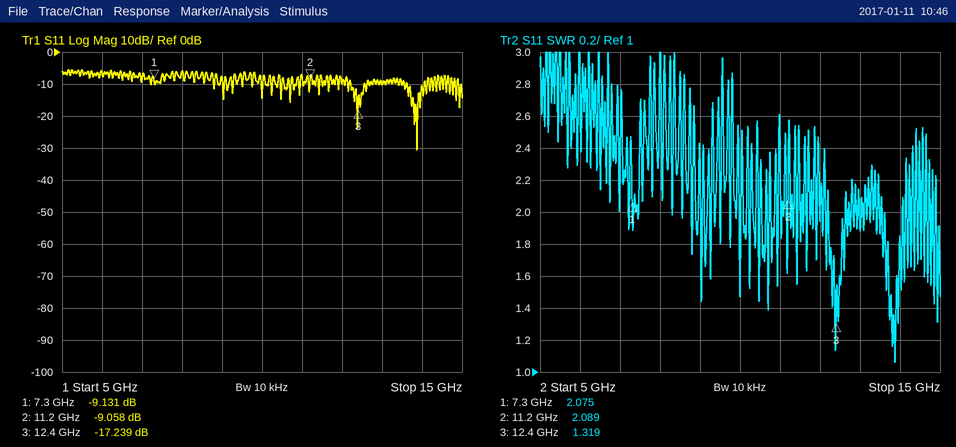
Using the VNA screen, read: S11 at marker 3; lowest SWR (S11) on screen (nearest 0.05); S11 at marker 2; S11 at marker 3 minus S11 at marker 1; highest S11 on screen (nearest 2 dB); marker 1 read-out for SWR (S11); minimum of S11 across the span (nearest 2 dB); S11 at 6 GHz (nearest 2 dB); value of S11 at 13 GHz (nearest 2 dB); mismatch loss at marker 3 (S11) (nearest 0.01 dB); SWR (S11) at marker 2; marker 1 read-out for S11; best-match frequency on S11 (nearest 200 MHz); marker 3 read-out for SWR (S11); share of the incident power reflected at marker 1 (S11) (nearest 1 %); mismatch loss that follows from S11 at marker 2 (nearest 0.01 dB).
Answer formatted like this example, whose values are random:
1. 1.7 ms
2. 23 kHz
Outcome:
1. -17.239 dB
2. 1.05
3. -9.058 dB
4. -8.108 dB
5. -6 dB
6. 2.075
7. -30 dB
8. -6 dB
9. -10 dB
10. 0.08 dB
11. 2.089
12. -9.131 dB
13. 13.8 GHz
14. 1.319
15. 12 %
16. 0.58 dB
